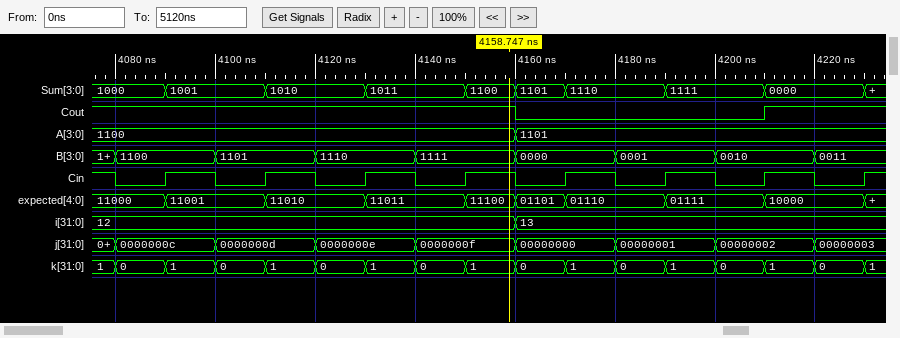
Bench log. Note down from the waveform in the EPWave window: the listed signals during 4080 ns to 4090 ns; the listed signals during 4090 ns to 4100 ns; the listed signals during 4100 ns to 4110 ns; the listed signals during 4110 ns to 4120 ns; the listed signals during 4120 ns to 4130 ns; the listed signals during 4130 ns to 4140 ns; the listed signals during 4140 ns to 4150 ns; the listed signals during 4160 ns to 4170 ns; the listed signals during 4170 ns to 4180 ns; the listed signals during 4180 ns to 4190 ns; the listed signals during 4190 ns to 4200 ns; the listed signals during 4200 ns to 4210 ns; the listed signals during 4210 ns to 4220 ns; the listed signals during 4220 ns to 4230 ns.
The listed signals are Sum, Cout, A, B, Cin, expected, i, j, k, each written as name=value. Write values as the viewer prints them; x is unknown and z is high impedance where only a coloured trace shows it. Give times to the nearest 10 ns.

Sum=1000, Cout=1, A=1100, B=1100, Cin=0, expected=11000, i=12, j=0000000c, k=0
Sum=1001, Cout=1, A=1100, B=1100, Cin=1, expected=11001, i=12, j=0000000c, k=1
Sum=1001, Cout=1, A=1100, B=1101, Cin=0, expected=11001, i=12, j=0000000d, k=0
Sum=1010, Cout=1, A=1100, B=1101, Cin=1, expected=11010, i=12, j=0000000d, k=1
Sum=1010, Cout=1, A=1100, B=1110, Cin=0, expected=11010, i=12, j=0000000e, k=0
Sum=1011, Cout=1, A=1100, B=1110, Cin=1, expected=11011, i=12, j=0000000e, k=1
Sum=1011, Cout=1, A=1100, B=1111, Cin=0, expected=11011, i=12, j=0000000f, k=0
Sum=1101, Cout=0, A=1101, B=0000, Cin=0, expected=01101, i=13, j=00000000, k=0
Sum=1110, Cout=0, A=1101, B=0000, Cin=1, expected=01110, i=13, j=00000000, k=1
Sum=1110, Cout=0, A=1101, B=0001, Cin=0, expected=01110, i=13, j=00000001, k=0
Sum=1111, Cout=0, A=1101, B=0001, Cin=1, expected=01111, i=13, j=00000001, k=1
Sum=1111, Cout=0, A=1101, B=0010, Cin=0, expected=01111, i=13, j=00000002, k=0
Sum=0000, Cout=1, A=1101, B=0010, Cin=1, expected=10000, i=13, j=00000002, k=1
Sum=0000, Cout=1, A=1101, B=0011, Cin=0, expected=10000, i=13, j=00000003, k=0
